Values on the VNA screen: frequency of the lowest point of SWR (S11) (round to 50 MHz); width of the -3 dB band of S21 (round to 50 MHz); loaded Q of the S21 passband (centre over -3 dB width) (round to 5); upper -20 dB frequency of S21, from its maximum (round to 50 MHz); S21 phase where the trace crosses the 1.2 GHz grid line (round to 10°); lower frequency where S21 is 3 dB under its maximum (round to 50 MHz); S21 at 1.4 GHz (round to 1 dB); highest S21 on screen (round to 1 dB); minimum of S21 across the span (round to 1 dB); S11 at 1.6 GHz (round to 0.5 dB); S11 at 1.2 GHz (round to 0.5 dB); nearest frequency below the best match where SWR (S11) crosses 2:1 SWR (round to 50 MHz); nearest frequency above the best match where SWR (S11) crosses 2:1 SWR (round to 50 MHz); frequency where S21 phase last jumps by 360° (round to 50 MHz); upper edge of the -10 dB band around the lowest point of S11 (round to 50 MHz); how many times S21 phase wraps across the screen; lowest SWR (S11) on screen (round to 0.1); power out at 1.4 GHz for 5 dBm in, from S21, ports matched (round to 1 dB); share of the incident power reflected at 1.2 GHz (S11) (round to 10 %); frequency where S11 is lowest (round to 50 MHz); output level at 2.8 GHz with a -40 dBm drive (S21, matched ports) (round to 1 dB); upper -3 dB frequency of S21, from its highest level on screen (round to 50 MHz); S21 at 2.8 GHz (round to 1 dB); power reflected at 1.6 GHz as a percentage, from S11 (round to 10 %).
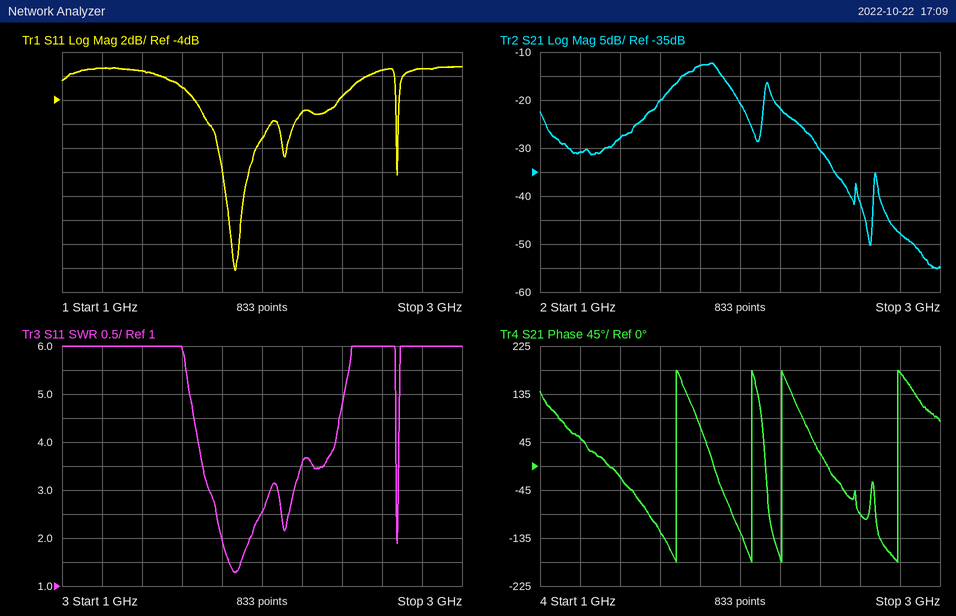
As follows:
1.85 GHz
200 MHz
10
2.45 GHz
50°
1.70 GHz
-28 dB
-12 dB
-55 dB
-3.0 dB
-1.5 dB
1.80 GHz
1.95 GHz
2.80 GHz
1.95 GHz
4
1.3
-23 dBm
70 %
1.85 GHz
-88 dBm
1.90 GHz
-48 dB
50 %
